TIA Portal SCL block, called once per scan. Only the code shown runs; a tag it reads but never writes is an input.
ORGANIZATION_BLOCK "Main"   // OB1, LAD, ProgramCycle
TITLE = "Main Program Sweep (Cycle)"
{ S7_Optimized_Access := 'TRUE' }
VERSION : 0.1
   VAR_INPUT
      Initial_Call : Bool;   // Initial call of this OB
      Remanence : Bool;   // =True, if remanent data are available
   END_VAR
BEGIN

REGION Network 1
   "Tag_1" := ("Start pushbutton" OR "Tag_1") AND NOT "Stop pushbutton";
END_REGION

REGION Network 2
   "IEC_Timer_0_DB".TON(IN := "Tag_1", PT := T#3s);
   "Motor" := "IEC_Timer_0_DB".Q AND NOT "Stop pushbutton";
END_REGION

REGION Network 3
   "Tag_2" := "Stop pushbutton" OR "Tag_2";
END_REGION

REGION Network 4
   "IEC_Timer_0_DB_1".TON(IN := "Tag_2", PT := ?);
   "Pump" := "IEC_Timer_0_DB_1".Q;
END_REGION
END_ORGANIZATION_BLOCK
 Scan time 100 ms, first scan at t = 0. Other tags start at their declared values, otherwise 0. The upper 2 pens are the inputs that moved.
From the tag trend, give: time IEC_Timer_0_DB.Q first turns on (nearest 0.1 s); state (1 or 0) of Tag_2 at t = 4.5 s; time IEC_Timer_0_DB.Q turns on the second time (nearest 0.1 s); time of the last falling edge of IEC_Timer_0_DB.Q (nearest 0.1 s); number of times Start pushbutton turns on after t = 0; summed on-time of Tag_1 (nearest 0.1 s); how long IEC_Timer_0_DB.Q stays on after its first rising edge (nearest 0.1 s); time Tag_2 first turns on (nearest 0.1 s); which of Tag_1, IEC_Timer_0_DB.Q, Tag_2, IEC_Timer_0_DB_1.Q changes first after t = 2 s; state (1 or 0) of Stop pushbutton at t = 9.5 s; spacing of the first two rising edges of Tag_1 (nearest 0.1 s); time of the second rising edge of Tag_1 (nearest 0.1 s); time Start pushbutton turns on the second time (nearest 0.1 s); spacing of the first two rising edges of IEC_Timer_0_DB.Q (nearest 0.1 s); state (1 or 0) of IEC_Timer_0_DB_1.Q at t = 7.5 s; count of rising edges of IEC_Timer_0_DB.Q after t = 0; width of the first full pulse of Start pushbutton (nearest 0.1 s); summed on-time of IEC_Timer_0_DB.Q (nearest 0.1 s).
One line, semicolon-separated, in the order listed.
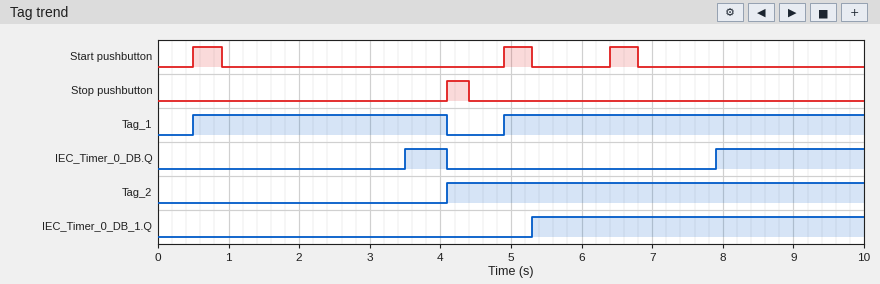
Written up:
3.5 s; 1; 7.9 s; 4.1 s; 3; 8.7 s; 0.6 s; 4.1 s; IEC_Timer_0_DB.Q; 0; 4.4 s; 4.9 s; 4.9 s; 4.4 s; 1; 2; 0.4 s; 2.7 s
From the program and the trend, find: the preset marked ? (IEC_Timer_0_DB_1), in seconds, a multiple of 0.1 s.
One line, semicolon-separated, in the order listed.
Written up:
1.2 s
